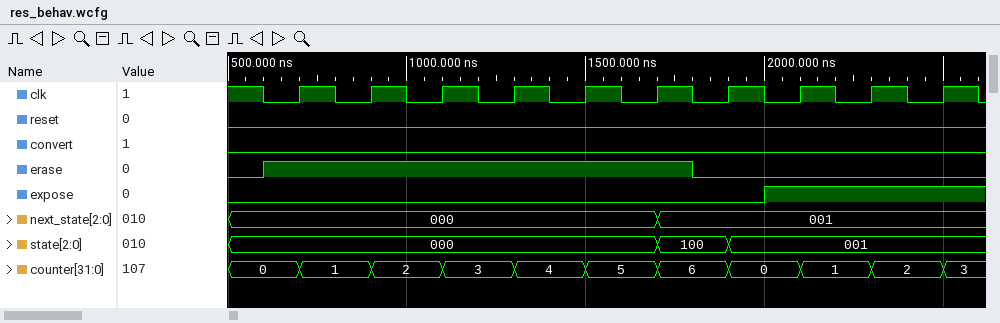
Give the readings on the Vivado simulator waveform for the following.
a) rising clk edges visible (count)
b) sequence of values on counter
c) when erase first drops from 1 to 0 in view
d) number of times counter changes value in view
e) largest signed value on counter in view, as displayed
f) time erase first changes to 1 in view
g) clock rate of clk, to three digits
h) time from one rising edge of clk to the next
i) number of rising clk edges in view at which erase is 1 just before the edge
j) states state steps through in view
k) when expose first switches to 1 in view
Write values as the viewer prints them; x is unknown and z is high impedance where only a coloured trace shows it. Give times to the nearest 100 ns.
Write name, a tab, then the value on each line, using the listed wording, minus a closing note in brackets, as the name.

rising clk edges visible	10
sequence of values on counter	0, 1, 2, 3, 4, 5, 6, 0, 1, 2, 3
when erase first drops from 1 to 0 in view	1800 ns
number of times counter changes value in view	10
largest signed value on counter in view, as displayed	6
time erase first changes to 1 in view	600 ns
clock rate of clk, to three digits	5.00 MHz
time from one rising edge of clk to the next	200 ns
number of rising clk edges in view at which erase is 1 just before the edge	6
states state steps through in view	000, 100, 001
when expose first switches to 1 in view	2000 ns
